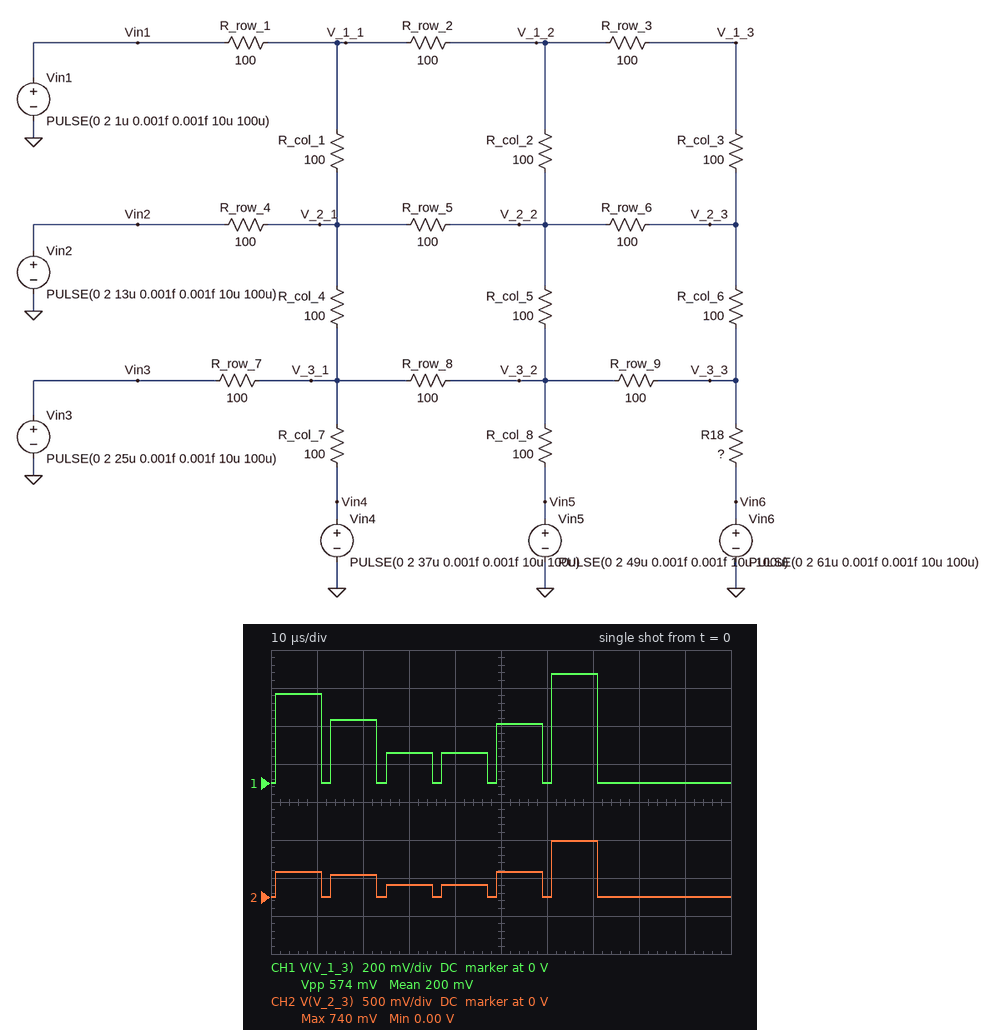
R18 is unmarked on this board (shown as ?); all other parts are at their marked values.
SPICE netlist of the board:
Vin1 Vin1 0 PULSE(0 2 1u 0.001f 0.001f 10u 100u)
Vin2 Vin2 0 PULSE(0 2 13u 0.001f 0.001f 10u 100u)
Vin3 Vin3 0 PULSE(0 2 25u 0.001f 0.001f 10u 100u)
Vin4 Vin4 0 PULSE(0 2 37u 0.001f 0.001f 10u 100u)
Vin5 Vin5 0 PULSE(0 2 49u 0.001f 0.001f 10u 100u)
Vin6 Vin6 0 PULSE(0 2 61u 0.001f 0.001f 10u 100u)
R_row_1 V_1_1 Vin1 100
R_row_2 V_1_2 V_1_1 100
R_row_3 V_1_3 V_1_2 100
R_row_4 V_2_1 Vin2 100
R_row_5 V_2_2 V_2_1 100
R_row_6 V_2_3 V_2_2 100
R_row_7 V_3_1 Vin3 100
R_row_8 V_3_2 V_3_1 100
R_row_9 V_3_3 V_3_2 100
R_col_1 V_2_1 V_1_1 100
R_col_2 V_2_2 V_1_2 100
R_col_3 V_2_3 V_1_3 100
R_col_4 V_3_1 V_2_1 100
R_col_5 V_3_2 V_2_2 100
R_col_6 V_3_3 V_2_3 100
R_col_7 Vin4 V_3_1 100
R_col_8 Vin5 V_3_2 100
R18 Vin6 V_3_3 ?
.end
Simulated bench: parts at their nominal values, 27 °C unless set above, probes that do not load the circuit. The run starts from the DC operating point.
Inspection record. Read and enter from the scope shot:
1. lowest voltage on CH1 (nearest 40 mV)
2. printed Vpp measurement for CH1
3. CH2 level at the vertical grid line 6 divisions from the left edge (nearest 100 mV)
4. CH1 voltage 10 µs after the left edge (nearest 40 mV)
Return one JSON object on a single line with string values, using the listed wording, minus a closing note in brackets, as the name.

{"lowest voltage on CH1": "0 V", "printed Vpp measurement for CH1": "574 mV", "CH2 level at the vertical grid line 6 divisions from the left edge": "0 V", "CH1 voltage 10 µs after the left edge": "480 mV"}
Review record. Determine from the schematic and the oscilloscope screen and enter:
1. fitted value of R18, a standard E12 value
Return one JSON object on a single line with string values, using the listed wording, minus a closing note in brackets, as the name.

{"fitted value of R18, a standard E12 value": "68 Ω"}
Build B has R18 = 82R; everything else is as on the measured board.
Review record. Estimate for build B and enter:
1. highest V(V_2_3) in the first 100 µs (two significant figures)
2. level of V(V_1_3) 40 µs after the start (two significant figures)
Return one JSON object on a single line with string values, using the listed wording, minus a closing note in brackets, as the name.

{"highest V(V_2_3) in the first 100 µs": "680 mV", "level of V(V_1_3) 40 µs after the start": "170 mV"}
